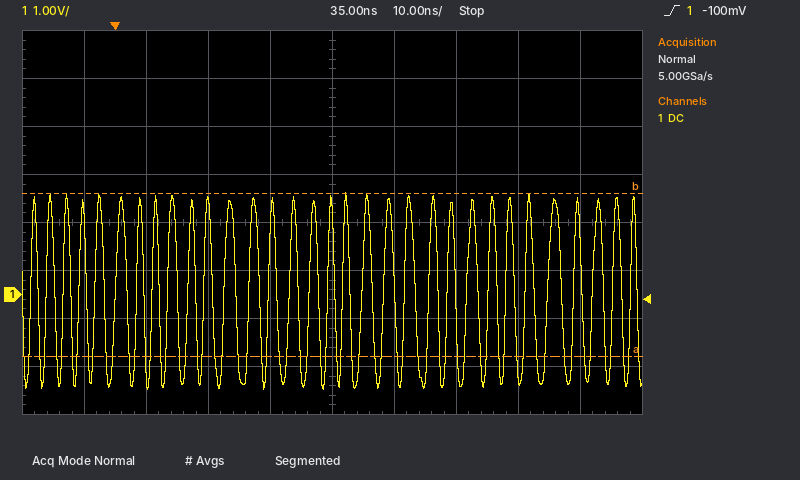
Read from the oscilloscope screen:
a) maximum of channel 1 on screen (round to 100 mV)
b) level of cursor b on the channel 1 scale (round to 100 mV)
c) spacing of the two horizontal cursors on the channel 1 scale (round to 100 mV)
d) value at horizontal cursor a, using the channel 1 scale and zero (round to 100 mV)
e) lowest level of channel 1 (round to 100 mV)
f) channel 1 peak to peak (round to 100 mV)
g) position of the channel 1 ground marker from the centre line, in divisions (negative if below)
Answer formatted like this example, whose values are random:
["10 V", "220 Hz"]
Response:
["2.1 V", "2.1 V", "3.4 V", "-1.3 V", "-2.0 V", "4.1 V", "-1.5 div"]
